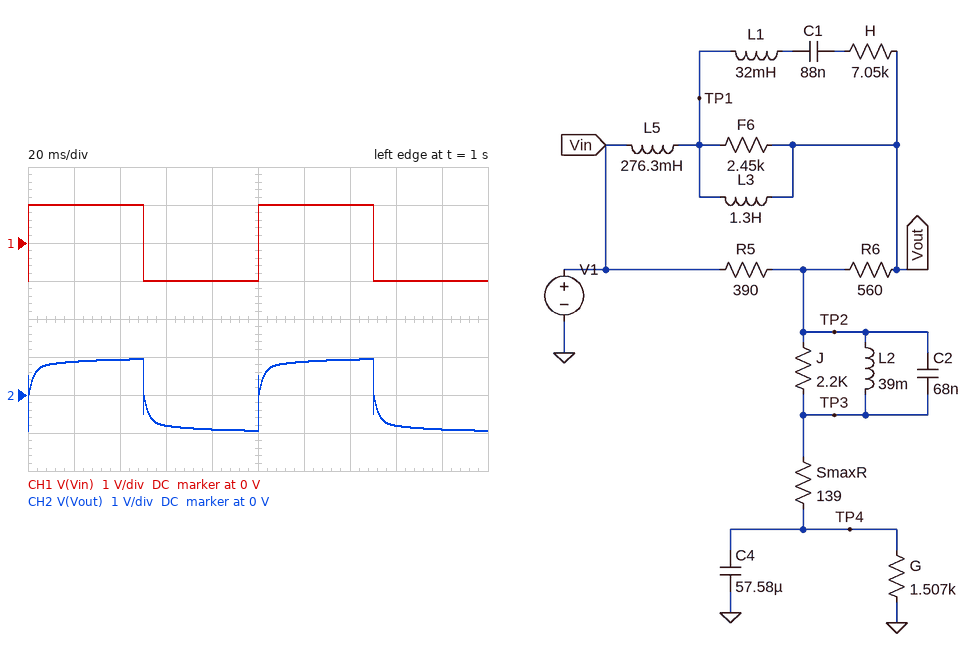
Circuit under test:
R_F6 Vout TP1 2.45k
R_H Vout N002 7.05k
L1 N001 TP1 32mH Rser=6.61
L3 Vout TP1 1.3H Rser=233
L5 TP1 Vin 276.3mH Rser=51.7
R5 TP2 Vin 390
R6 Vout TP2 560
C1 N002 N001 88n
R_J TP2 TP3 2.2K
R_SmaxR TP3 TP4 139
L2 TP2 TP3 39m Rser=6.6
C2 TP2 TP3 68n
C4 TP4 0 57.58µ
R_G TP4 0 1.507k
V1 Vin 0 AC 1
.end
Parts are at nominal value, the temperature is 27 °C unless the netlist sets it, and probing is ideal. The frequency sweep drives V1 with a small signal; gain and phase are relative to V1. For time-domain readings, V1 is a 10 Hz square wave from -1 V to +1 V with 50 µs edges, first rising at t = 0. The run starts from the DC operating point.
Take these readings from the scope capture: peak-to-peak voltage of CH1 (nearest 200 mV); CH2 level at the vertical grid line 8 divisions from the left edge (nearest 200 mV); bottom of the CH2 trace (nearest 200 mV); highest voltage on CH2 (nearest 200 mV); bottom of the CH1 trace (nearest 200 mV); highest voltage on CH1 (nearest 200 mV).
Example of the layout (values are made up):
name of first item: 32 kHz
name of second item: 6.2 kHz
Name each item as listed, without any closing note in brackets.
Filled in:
peak-to-peak voltage of CH1: 2.0 V
CH2 level at the vertical grid line 8 divisions from the left edge: -800 mV
bottom of the CH2 trace: -1.0 V
highest voltage on CH2: 1.0 V
bottom of the CH1 trace: -1.0 V
highest voltage on CH1: 1.0 V
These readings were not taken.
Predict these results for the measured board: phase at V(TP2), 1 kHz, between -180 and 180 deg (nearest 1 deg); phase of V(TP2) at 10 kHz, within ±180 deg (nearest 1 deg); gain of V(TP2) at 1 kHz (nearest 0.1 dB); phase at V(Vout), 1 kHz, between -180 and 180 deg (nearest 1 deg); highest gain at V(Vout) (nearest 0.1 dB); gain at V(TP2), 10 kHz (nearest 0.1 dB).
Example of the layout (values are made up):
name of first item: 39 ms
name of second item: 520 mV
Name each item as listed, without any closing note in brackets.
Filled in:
phase at V(TP2), 1 kHz, between -180 and 180 deg: 27 deg
phase of V(TP2) at 10 kHz, within ±180 deg: -33 deg
gain of V(TP2) at 1 kHz: -5.6 dB
phase at V(Vout), 1 kHz, between -180 and 180 deg: 16 deg
highest gain at V(Vout): -0.4 dB
gain at V(TP2), 10 kHz: -6.0 dB
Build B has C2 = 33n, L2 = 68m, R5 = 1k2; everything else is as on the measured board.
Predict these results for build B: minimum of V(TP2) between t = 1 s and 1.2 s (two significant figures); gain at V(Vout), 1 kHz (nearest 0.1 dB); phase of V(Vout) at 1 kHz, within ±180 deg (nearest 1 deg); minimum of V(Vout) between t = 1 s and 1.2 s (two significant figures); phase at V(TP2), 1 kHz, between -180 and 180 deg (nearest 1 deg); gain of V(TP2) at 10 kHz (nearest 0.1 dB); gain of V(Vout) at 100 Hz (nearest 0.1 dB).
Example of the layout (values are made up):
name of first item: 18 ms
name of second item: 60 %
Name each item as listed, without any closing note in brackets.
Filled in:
minimum of V(TP2) between t = 1 s and 1.2 s: -640 mV
gain at V(Vout), 1 kHz: -7.8 dB
phase of V(Vout) at 1 kHz, within ±180 deg: 15 deg
minimum of V(Vout) between t = 1 s and 1.2 s: -890 mV
phase at V(TP2), 1 kHz, between -180 and 180 deg: 33 deg
gain of V(TP2) at 10 kHz: -8.4 dB
gain of V(Vout) at 100 Hz: -5.7 dB
